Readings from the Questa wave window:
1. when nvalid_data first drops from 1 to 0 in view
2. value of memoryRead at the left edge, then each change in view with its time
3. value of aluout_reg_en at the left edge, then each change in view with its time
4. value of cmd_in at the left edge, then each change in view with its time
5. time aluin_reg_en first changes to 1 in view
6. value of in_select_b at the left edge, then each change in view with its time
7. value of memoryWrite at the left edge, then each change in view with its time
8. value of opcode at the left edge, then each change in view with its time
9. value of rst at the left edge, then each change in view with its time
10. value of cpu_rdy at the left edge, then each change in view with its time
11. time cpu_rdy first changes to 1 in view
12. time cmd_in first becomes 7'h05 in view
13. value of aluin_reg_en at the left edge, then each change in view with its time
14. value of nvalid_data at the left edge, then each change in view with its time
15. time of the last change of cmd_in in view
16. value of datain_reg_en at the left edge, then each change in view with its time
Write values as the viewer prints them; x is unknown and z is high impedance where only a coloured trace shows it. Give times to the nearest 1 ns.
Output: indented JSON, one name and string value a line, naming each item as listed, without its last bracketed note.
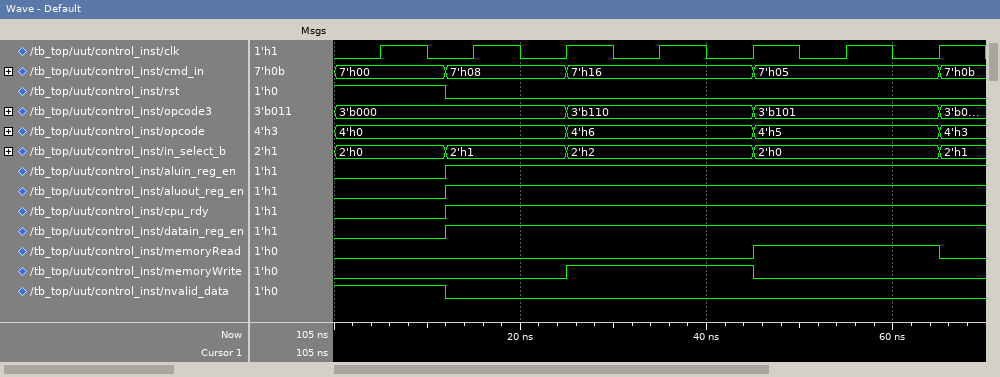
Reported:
{
  "when nvalid_data first drops from 1 to 0 in view": "12 ns",
  "value of memoryRead at the left edge, then each change in view with its time": "0, 1 at 45 ns, 0 at 65 ns",
  "value of aluout_reg_en at the left edge, then each change in view with its time": "0, 1 at 12 ns",
  "value of cmd_in at the left edge, then each change in view with its time": "7'h00, 7'h08 at 12 ns, 7'h16 at 25 ns, 7'h05 at 45 ns, 7'h0b at 65 ns",
  "time aluin_reg_en first changes to 1 in view": "12 ns",
  "value of in_select_b at the left edge, then each change in view with its time": "2'h0, 2'h1 at 12 ns, 2'h2 at 25 ns, 2'h0 at 45 ns, 2'h1 at 65 ns",
  "value of memoryWrite at the left edge, then each change in view with its time": "0, 1 at 25 ns, 0 at 45 ns",
  "value of opcode at the left edge, then each change in view with its time": "4'h0, 4'h6 at 25 ns, 4'h5 at 45 ns, 4'h3 at 65 ns",
  "value of rst at the left edge, then each change in view with its time": "1, 0 at 12 ns",
  "value of cpu_rdy at the left edge, then each change in view with its time": "0, 1 at 12 ns",
  "time cpu_rdy first changes to 1 in view": "12 ns",
  "time cmd_in first becomes 7'h05 in view": "45 ns",
  "value of aluin_reg_en at the left edge, then each change in view with its time": "0, 1 at 12 ns",
  "value of nvalid_data at the left edge, then each change in view with its time": "1, 0 at 12 ns",
  "time of the last change of cmd_in in view": "65 ns",
  "value of datain_reg_en at the left edge, then each change in view with its time": "0, 1 at 12 ns"
}
